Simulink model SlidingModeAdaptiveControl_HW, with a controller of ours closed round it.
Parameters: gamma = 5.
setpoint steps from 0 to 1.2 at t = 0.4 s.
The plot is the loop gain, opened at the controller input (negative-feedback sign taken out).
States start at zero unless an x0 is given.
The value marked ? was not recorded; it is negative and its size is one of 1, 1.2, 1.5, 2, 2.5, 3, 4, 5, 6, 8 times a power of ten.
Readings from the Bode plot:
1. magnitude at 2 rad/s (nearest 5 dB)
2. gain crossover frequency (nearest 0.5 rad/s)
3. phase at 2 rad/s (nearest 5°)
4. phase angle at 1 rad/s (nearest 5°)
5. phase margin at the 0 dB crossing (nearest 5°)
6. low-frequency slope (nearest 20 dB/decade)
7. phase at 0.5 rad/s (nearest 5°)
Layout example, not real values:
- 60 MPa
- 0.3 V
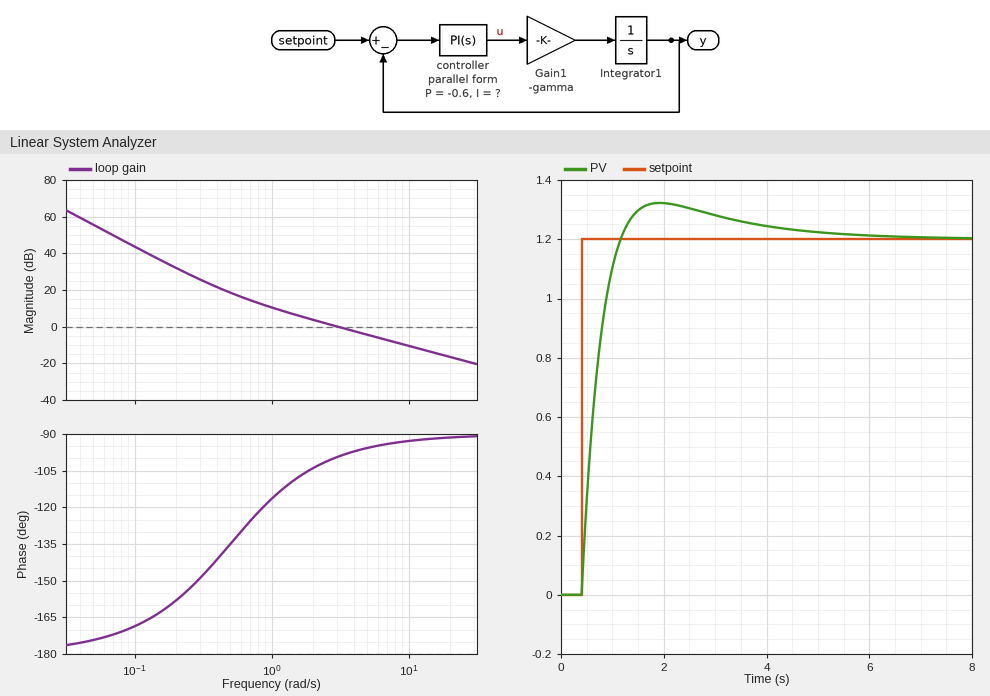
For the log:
- 5 dB
- 3.0 rad/s
- -105°
- -115°
- 80°
- -40 dB/decade
- -135°
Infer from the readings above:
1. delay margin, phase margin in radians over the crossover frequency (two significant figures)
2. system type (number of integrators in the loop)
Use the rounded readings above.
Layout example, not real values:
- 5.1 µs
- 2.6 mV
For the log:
- 0.47 s
- 2
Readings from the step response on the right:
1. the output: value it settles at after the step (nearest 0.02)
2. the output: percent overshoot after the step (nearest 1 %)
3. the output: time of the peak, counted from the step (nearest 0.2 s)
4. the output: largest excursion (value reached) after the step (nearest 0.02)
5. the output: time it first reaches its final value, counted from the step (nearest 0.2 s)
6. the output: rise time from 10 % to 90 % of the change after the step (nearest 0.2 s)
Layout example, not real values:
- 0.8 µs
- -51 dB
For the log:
- 1.20
- 10 %
- 1.6 s
- 1.32
- 0.8 s
- 0.6 s
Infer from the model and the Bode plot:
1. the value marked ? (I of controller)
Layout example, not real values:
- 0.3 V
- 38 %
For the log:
- -0.3
